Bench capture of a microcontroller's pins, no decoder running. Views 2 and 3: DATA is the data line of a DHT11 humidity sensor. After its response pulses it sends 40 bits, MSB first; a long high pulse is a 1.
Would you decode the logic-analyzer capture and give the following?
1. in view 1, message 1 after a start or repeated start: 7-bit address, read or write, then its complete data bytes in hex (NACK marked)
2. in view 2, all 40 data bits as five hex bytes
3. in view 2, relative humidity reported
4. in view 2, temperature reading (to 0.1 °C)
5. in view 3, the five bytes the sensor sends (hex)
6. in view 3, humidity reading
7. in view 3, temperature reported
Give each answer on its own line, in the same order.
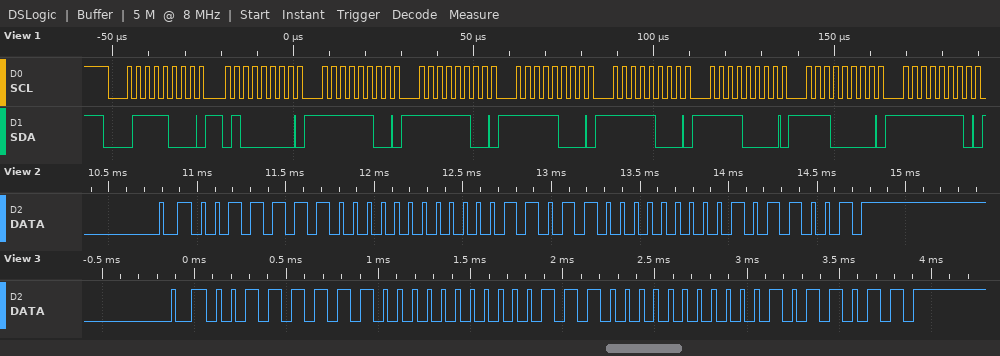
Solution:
0x3C write: 40 FC FC F8 F8 F0 E0 FE
3E 00 1B 00 59
62 %
27.0 °C
3F 00 1C 00 5B
63 %
28.0 °C
